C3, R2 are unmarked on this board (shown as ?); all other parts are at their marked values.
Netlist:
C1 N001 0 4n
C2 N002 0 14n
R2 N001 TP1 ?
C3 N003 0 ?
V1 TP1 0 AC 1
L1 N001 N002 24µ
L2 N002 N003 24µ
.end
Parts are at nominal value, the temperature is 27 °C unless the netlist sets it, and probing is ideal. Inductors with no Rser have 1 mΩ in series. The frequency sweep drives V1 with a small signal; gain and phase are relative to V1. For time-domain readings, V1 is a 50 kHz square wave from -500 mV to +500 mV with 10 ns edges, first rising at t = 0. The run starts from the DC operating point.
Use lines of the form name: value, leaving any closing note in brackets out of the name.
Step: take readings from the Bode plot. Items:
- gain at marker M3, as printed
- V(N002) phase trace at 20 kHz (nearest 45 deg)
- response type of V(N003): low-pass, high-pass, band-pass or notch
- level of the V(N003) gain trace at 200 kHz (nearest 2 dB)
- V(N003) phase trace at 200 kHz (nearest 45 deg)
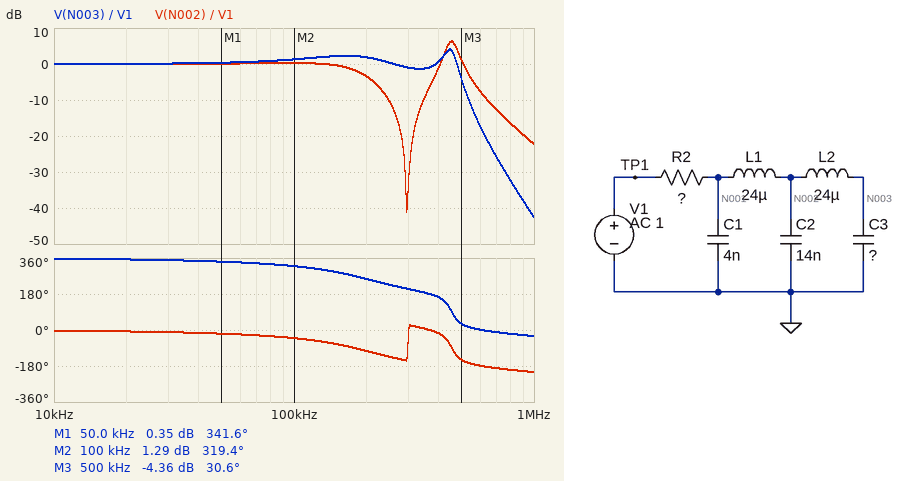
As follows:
gain at marker M3, as printed: -4.36 dB
V(N002) phase trace at 20 kHz: 0 deg
response type of V(N003): low-pass, high-pass, band-pass or notch: low-pass
level of the V(N003) gain trace at 200 kHz: 2 dB
V(N003) phase trace at 200 kHz: 270 deg
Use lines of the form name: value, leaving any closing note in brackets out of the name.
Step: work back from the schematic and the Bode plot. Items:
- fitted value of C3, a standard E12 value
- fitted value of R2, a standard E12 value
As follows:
fitted value of C3, a standard E12 value: 12 nF
fitted value of R2, a standard E12 value: 33 Ω
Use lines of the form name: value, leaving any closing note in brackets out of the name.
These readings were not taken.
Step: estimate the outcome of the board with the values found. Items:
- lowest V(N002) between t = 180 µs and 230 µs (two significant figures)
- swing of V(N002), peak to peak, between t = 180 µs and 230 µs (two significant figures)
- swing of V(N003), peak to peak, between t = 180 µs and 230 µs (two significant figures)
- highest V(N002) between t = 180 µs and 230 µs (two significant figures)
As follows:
lowest V(N002) between t = 180 µs and 230 µs: -820 mV
swing of V(N002), peak to peak, between t = 180 µs and 230 µs: 1.6 V
swing of V(N003), peak to peak, between t = 180 µs and 230 µs: 1.6 V
highest V(N002) between t = 180 µs and 230 µs: 820 mV
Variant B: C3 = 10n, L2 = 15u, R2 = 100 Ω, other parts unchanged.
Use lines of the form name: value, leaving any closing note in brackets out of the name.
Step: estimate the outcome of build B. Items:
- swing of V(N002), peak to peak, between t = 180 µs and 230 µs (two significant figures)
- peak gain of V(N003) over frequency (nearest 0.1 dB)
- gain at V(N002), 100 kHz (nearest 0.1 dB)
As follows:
swing of V(N002), peak to peak, between t = 180 µs and 230 µs: 970 mV
peak gain of V(N003) over frequency: 0 dB
gain at V(N002), 100 kHz: -5.6 dB
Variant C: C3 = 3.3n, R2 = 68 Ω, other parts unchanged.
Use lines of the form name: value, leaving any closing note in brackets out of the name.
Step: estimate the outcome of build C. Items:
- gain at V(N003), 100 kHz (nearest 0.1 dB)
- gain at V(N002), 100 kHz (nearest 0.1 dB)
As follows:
gain at V(N003), 100 kHz: -1.4 dB
gain at V(N002), 100 kHz: -1.7 dB
